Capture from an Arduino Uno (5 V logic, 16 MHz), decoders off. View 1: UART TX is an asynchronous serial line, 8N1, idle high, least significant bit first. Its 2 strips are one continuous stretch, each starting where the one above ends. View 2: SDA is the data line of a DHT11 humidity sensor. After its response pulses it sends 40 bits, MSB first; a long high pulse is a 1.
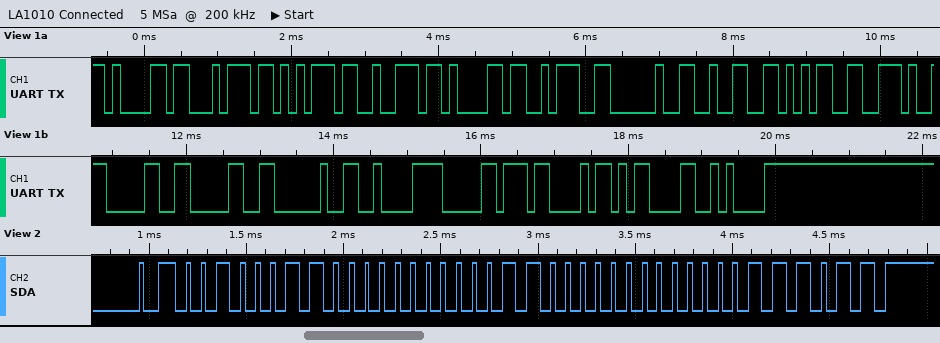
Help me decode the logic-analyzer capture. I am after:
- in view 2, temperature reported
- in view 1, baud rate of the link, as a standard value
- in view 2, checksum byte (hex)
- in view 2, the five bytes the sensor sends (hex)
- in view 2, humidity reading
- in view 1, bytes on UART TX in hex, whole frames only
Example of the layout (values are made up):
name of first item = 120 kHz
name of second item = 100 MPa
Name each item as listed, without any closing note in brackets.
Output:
in view 2, temperature reported = 24.0 °C
in view 1, baud rate of the link, as a standard value = 9600 baud
in view 2, checksum byte = 0x3B
in view 2, the five bytes the sensor sends = 23 00 18 00 3B
in view 2, humidity reading = 35 %
in view 1, bytes on UART TX in hex, whole frames only = 61 74 75 72 61 3A 20 32 35 2E 30 30 20 C2 B0 43 0D 0A
